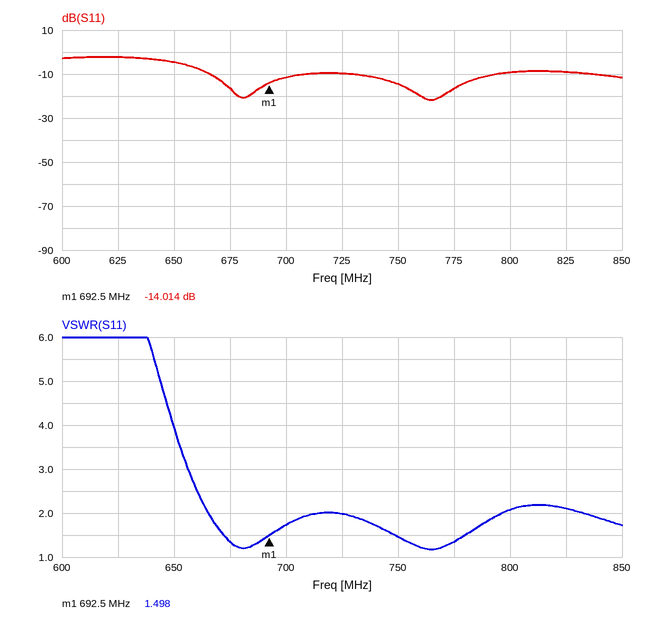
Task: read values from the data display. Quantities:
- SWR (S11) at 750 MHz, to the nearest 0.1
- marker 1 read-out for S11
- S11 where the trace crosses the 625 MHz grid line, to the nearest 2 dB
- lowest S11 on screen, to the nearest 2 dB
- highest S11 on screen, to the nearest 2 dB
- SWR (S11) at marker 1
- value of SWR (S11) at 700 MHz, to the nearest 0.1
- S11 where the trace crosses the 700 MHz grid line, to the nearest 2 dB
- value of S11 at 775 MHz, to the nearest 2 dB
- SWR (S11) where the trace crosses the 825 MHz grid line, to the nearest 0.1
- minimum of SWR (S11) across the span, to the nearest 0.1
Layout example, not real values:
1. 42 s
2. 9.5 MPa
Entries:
1. 1.5
2. -14.014 dB
3. -2 dB
4. -22 dB
5. -2 dB
6. 1.498
7. 1.7
8. -12 dB
9. -16 dB
10. 2.1
11. 1.2
